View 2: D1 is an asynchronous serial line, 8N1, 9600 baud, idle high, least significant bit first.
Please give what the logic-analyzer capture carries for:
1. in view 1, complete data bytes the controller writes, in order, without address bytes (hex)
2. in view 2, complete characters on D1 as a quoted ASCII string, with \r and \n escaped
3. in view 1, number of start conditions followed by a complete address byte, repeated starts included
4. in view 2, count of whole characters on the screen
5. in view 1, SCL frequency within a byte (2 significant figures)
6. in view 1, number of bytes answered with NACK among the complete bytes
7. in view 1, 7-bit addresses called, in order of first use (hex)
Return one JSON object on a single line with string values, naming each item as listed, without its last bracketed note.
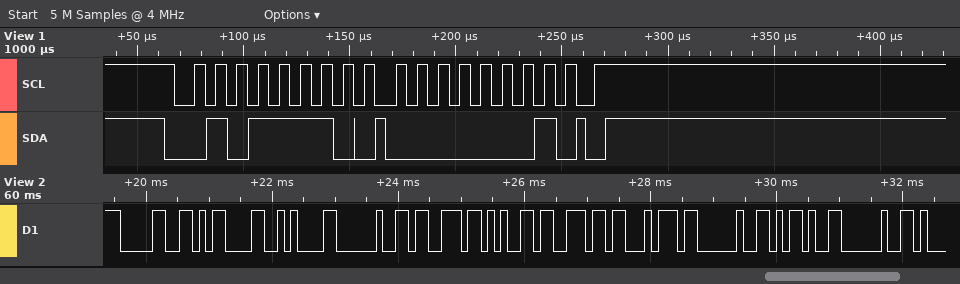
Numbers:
{"in view 1, complete data bytes the controller writes, in order, without address bytes": "01", "in view 2, complete characters on D1 as a quoted ASCII string, with \\r and \\n escaped": "\"0\\r\\n sent - \"", "in view 1, number of start conditions followed by a complete address byte, repeated starts included": "1", "in view 2, count of whole characters on the screen": "11", "in view 1, SCL frequency within a byte": "100 kHz", "in view 1, number of bytes answered with NACK among the complete bytes": "0", "in view 1, 7-bit addresses called, in order of first use": "0x2F"}
